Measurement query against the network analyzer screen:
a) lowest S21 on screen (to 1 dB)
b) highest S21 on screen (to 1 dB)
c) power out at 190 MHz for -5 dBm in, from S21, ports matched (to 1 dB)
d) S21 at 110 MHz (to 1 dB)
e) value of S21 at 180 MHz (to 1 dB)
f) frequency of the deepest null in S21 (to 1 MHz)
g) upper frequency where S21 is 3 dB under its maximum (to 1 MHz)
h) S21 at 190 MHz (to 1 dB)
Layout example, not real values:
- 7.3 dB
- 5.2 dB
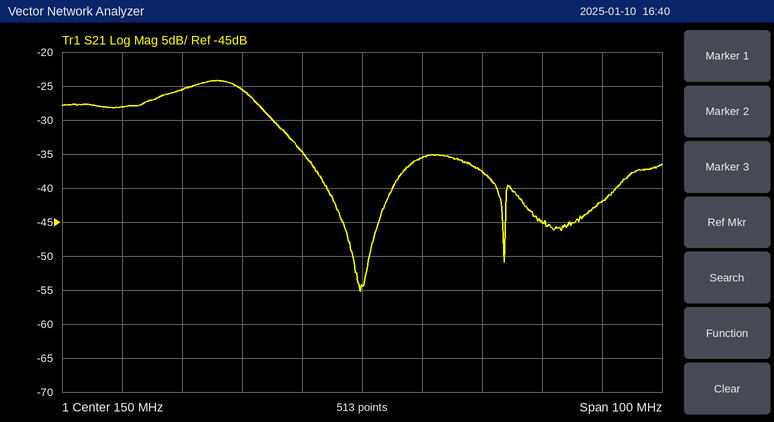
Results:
- -55 dB
- -24 dB
- -47 dBm
- -28 dB
- -45 dB
- 150 MHz
- 132 MHz
- -42 dB
